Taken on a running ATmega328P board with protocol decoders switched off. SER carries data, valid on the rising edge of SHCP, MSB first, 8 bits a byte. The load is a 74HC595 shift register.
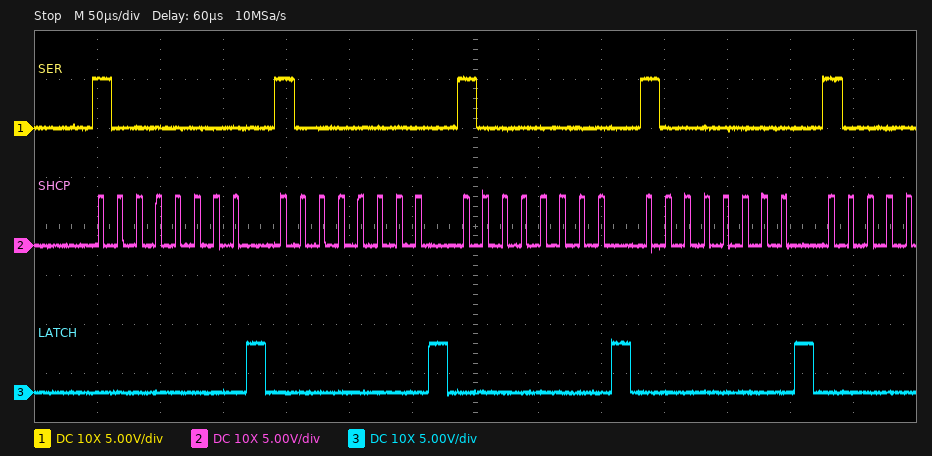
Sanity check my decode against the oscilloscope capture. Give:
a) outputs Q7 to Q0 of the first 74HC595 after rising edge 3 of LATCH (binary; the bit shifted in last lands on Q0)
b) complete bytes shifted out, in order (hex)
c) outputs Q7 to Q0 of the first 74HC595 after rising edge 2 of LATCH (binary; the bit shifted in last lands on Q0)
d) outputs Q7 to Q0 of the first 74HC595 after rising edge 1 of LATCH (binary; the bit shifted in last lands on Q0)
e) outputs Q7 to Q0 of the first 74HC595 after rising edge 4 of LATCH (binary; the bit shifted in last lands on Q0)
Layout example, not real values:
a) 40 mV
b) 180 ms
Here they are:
a) 10000000
b) 80 80 80 80
c) 10000000
d) 10000000
e) 10000000
